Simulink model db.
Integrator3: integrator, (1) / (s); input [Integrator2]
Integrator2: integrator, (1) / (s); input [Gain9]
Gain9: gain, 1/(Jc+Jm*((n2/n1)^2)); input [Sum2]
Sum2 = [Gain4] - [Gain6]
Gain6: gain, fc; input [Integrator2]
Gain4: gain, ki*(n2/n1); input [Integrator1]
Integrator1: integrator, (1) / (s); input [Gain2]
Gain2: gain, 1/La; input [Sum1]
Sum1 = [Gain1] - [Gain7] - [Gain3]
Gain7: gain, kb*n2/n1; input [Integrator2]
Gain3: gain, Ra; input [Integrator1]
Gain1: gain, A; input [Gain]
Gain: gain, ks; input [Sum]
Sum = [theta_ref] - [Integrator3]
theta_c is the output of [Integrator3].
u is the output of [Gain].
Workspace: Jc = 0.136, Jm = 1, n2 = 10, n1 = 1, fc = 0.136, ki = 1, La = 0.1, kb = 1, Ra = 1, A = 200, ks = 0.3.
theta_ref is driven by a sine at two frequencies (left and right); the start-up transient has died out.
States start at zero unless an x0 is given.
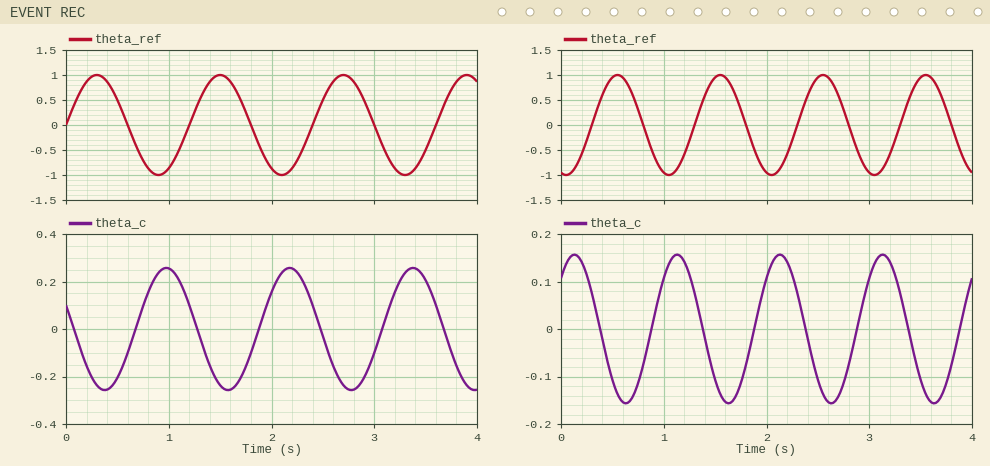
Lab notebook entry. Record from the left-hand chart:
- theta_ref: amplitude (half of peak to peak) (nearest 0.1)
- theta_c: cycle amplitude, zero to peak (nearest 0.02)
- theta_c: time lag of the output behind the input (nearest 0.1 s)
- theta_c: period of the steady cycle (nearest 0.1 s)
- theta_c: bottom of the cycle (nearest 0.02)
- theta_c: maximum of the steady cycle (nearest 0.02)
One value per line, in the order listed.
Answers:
1.0
0.26
0.7 s
1.2 s
-0.26
0.26
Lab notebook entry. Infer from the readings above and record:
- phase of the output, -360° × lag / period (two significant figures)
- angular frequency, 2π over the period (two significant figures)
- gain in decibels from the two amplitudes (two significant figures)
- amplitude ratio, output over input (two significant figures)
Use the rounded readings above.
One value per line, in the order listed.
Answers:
-210°
5.2 rad/s
-12 dB
0.26
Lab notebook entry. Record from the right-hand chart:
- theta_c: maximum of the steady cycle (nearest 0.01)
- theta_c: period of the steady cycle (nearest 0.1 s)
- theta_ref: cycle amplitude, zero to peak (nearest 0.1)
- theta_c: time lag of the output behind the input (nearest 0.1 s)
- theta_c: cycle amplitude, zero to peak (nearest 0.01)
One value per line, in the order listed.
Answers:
0.16
1.0 s
1.0
0.6 s
0.16
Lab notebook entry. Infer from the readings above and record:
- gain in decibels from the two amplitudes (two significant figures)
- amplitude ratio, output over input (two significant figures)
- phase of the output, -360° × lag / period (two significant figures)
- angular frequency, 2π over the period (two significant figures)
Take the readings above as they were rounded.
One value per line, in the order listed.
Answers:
-16 dB
0.16
-220°
6.3 rad/s
